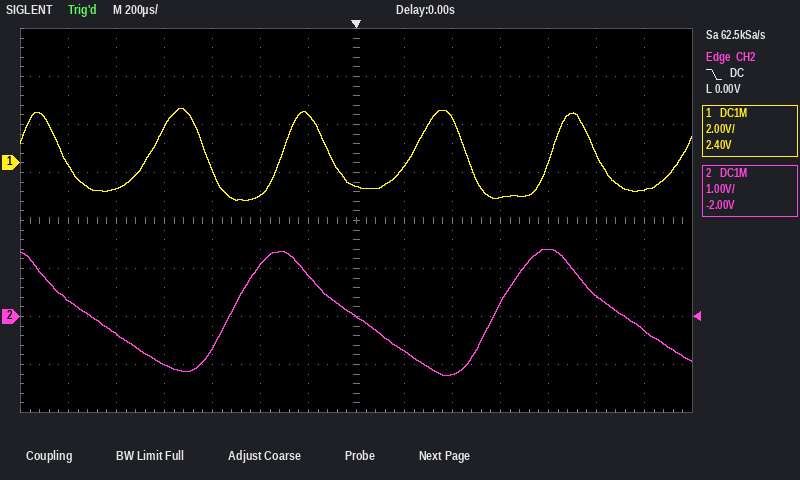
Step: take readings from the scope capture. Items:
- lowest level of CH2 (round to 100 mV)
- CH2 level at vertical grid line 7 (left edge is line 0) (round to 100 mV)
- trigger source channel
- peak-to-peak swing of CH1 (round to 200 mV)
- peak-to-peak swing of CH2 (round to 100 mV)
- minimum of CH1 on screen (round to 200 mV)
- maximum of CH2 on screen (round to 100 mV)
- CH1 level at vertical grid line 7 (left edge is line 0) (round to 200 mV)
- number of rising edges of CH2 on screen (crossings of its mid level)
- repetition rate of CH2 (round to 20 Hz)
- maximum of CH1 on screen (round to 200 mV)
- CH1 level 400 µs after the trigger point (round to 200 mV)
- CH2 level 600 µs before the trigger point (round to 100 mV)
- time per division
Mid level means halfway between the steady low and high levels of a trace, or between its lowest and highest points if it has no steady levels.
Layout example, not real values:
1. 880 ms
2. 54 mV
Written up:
1. -1.2 V
2. 0.0 V
3. CH2
4. 3.8 V
5. 2.6 V
6. -1.6 V
7. 1.4 V
8. -1.0 V
9. 2
10. 900 Hz
11. 2.2 V
12. 1.8 V
13. -700 mV
14. 200 µs
